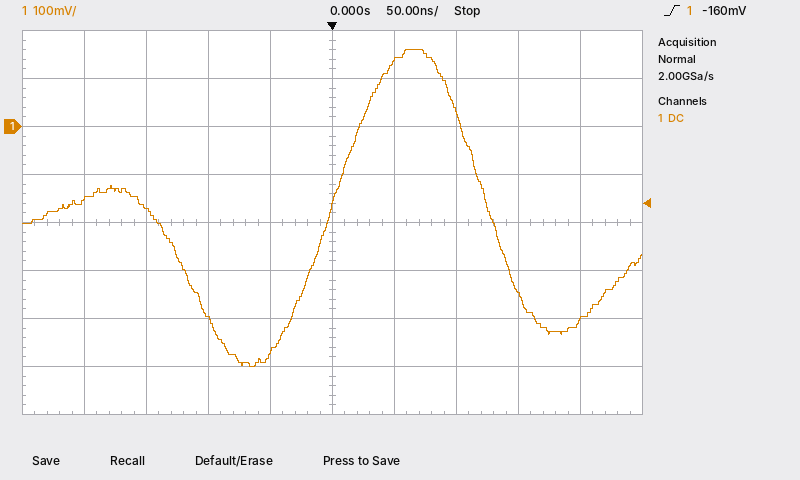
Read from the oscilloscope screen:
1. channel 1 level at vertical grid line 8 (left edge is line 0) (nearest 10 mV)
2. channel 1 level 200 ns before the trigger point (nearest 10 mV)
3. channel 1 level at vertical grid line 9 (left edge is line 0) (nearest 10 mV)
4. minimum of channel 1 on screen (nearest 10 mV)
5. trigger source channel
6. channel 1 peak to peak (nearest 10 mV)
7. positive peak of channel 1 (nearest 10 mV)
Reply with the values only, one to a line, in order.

-350 mV
-150 mV
-400 mV
-500 mV
channel 1
660 mV
160 mV
